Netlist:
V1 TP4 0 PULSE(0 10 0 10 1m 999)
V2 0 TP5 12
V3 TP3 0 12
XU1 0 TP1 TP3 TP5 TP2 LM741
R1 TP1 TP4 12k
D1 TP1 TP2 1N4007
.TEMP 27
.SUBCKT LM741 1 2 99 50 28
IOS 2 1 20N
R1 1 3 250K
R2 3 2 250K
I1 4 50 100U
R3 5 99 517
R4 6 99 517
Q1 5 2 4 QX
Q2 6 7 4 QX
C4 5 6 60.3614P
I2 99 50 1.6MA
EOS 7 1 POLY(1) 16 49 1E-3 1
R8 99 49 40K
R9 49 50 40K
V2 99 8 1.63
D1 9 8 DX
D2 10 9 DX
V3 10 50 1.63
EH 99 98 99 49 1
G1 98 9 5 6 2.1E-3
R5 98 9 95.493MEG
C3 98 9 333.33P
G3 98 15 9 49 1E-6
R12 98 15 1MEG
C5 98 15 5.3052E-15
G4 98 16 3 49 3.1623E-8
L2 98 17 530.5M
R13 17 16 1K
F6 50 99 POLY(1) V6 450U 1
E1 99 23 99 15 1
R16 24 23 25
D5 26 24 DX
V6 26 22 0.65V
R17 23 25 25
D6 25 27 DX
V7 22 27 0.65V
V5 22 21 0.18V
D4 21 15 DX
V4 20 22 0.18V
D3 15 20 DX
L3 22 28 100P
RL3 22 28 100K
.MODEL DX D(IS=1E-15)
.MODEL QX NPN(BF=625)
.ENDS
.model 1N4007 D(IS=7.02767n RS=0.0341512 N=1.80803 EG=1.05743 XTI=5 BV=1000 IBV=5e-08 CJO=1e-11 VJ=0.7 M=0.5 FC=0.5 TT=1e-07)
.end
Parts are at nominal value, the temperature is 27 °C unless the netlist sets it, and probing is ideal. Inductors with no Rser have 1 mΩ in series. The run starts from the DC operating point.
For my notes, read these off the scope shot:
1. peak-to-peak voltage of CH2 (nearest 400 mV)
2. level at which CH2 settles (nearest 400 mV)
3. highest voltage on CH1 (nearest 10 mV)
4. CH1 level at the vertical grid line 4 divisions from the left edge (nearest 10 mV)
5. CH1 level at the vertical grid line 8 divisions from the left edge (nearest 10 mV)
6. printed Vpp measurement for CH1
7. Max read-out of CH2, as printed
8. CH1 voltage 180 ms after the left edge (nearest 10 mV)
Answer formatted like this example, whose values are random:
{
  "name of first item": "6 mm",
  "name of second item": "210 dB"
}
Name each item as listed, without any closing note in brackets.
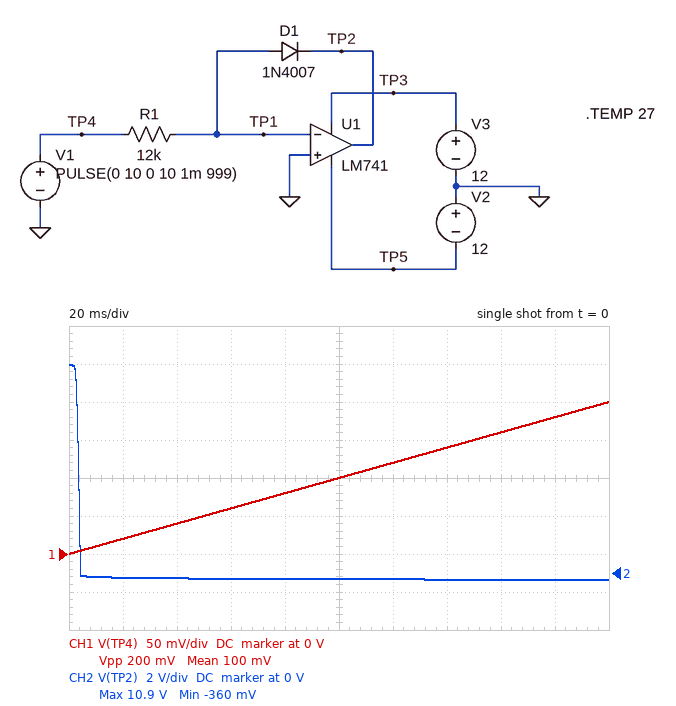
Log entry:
{
  "peak-to-peak voltage of CH2": "11.2 V",
  "level at which CH2 settles": "-400 mV",
  "highest voltage on CH1": "200 mV",
  "CH1 level at the vertical grid line 4 divisions from the left edge": "80 mV",
  "CH1 level at the vertical grid line 8 divisions from the left edge": "160 mV",
  "printed Vpp measurement for CH1": "200 mV",
  "Max read-out of CH2, as printed": "10.9 V",
  "CH1 voltage 180 ms after the left edge": "180 mV"
}
